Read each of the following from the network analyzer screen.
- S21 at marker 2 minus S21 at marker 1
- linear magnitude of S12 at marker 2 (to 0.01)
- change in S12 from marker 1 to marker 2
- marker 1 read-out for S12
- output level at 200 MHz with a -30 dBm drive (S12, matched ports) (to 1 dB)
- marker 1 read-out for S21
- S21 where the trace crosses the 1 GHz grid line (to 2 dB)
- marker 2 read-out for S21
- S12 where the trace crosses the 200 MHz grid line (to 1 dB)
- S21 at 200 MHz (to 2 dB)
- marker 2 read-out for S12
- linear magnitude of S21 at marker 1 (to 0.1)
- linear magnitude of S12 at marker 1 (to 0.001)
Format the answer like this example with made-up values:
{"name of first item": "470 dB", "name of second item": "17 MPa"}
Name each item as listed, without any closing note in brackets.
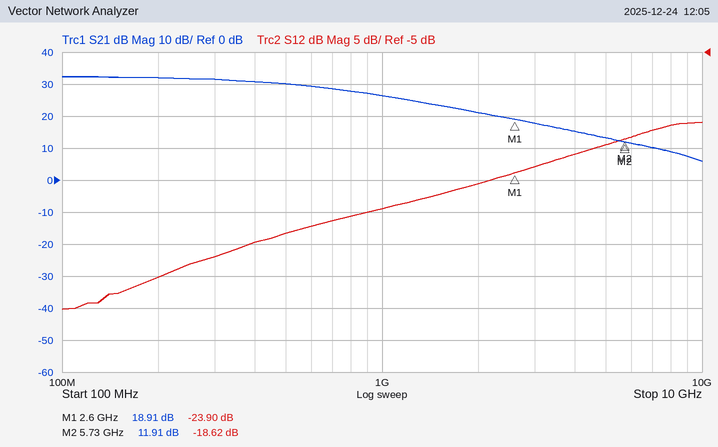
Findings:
{"S21 at marker 2 minus S21 at marker 1": "-7.00 dB", "linear magnitude of S12 at marker 2": "0.12", "change in S12 from marker 1 to marker 2": "5.28 dB", "marker 1 read-out for S12": "-23.90 dB", "output level at 200 MHz with a -30 dBm drive (S12, matched ports)": "-70 dBm", "marker 1 read-out for S21": "18.91 dB", "S21 where the trace crosses the 1 GHz grid line": "26 dB", "marker 2 read-out for S21": "11.91 dB", "S12 where the trace crosses the 200 MHz grid line": "-40 dB", "S21 at 200 MHz": "32 dB", "marker 2 read-out for S12": "-18.62 dB", "linear magnitude of S21 at marker 1": "8.8", "linear magnitude of S12 at marker 1": "0.064"}
